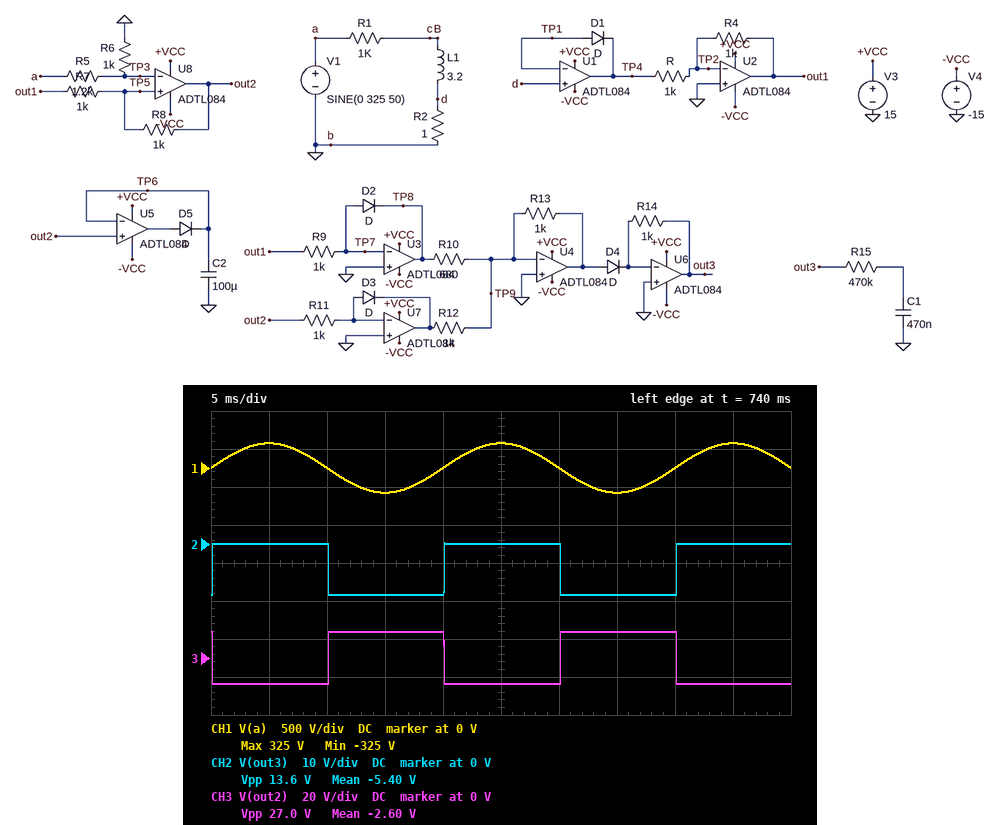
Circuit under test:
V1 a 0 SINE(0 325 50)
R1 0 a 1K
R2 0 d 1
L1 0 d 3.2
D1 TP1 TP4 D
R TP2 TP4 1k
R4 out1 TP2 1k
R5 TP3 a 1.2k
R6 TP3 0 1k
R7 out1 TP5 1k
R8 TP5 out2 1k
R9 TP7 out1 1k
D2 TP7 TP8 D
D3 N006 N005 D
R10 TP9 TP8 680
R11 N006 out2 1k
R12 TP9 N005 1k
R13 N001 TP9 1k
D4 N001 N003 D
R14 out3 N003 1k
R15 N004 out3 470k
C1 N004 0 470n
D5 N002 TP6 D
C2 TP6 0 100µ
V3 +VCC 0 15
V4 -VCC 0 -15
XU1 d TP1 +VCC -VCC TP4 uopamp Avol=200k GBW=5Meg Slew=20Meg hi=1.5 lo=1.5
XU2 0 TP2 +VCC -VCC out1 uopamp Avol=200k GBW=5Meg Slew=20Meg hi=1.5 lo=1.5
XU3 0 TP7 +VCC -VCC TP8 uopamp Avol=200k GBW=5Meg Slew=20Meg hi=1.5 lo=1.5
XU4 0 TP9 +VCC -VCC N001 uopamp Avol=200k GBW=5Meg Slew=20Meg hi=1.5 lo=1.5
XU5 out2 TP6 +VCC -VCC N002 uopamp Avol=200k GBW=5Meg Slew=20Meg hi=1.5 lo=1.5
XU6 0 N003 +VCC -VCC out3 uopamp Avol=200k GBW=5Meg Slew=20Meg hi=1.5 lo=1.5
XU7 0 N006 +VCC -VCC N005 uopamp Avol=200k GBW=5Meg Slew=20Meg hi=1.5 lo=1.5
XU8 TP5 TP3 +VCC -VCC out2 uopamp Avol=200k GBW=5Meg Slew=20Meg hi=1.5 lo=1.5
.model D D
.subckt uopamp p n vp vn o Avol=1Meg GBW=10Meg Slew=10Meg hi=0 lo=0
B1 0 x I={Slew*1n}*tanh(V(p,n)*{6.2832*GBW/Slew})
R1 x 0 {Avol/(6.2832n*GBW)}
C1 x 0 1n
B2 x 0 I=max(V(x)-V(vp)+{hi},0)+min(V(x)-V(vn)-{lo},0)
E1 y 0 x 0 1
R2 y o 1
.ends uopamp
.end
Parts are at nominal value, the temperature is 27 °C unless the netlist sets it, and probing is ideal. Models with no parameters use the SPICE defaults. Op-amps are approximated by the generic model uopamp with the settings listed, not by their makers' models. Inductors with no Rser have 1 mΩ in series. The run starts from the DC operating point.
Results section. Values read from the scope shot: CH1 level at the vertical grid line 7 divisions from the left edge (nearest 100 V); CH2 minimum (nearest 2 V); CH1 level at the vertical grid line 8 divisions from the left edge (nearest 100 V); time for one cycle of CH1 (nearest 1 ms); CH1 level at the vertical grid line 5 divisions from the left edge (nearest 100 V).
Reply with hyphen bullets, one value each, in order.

- -300 V
- -14 V
- 0 V
- 20 ms
- 300 V
